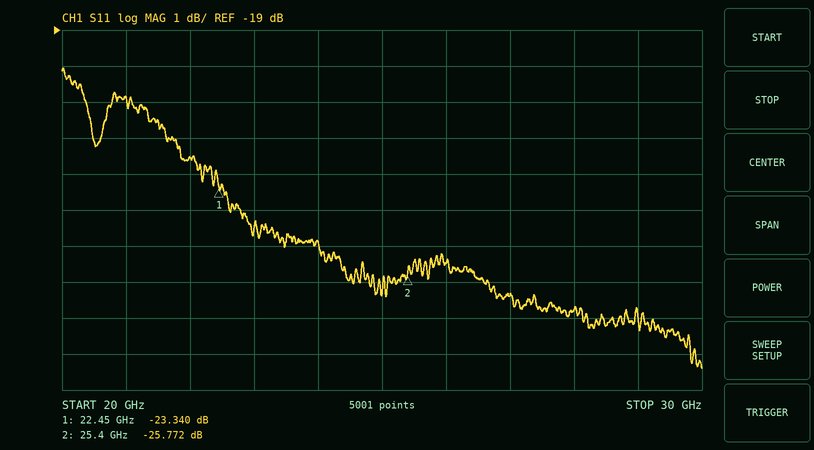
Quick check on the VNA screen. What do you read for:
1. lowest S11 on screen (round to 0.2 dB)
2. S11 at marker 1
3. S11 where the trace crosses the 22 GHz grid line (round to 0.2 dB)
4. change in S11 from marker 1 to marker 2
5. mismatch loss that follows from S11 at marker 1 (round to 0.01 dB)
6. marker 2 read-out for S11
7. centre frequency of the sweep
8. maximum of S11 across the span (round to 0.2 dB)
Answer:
-28.4 dB
-23.340 dB
-22.6 dB
-2.432 dB
0.02 dB
-25.772 dB
25 GHz
-20.0 dB
